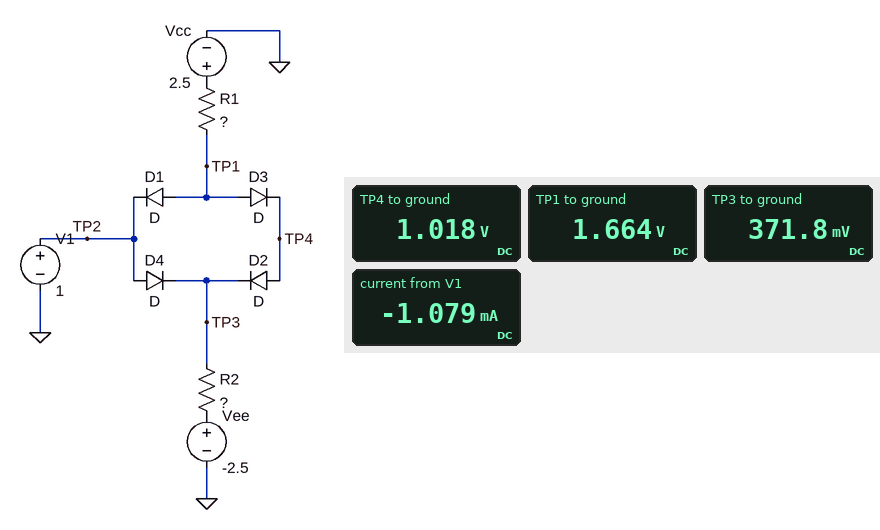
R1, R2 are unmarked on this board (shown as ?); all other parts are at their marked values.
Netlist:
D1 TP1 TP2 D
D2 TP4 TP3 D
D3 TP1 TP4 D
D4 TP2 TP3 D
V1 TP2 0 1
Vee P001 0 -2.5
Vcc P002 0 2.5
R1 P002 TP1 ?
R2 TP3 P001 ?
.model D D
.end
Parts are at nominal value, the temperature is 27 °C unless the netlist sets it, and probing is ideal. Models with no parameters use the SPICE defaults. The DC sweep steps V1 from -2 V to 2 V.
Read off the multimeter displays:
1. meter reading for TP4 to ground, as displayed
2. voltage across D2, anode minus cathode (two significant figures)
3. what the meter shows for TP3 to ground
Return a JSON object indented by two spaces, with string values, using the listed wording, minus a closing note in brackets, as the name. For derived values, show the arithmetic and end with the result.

{
  "meter reading for TP4 to ground, as displayed": "1.018 V",
  "voltage across D2, anode minus cathode": "1.018 V - 371.8 mV = 650 mV",
  "what the meter shows for TP3 to ground": "371.8 mV"
}
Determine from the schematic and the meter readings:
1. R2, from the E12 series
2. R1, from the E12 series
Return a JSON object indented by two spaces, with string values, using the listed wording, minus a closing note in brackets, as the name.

{
  "R2, from the E12 series": "2.7 kΩ",
  "R1, from the E12 series": "390 Ω"
}
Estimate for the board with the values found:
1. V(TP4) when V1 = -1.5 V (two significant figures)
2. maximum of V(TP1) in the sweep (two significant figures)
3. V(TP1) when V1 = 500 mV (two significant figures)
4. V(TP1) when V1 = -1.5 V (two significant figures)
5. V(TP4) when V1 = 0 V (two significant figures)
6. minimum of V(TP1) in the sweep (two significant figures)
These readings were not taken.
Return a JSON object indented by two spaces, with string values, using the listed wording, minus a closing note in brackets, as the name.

{
  "V(TP4) when V1 = -1.5 V": "-1.4 V",
  "maximum of V(TP1) in the sweep": "2.5 V",
  "V(TP1) when V1 = 500 mV": "1.2 V",
  "V(TP1) when V1 = -1.5 V": "-790 mV",
  "V(TP4) when V1 = 0 V": "49 mV",
  "minimum of V(TP1) in the sweep": "-1.3 V"
}
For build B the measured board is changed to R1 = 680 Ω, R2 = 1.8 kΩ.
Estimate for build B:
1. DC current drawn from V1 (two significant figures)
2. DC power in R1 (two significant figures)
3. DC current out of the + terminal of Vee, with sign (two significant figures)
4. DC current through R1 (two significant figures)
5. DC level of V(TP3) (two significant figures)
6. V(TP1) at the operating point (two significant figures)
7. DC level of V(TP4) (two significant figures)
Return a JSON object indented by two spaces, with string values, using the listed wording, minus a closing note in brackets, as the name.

{
  "DC current drawn from V1": "320 µA",
  "DC power in R1": "1.1 mW",
  "DC current out of the + terminal of Vee, with sign": "-1.6 mA",
  "DC current through R1": "1.3 mA",
  "DC level of V(TP3)": "350 mV",
  "V(TP1) at the operating point": "1.6 V",
  "DC level of V(TP4)": "990 mV"
}
